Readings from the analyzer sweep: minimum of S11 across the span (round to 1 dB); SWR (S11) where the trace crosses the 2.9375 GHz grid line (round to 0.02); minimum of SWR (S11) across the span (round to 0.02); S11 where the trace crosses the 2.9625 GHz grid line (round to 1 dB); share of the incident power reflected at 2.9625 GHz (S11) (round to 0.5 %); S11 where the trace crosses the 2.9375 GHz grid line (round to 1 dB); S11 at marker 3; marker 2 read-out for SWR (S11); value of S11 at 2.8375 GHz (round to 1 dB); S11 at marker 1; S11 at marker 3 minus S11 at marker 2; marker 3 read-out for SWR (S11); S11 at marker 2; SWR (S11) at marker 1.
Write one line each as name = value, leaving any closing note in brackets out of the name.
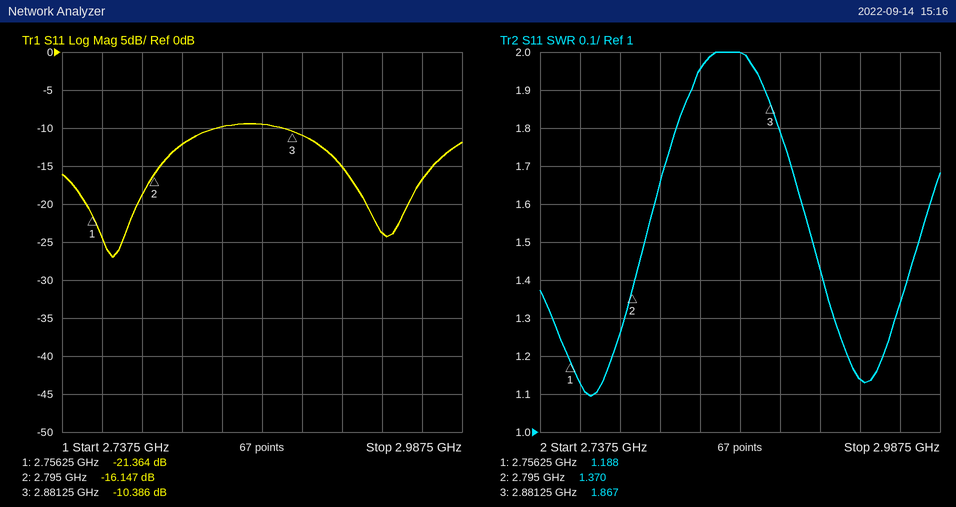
minimum of S11 across the span = -27 dB
SWR (S11) where the trace crosses the 2.9375 GHz grid line = 1.14
minimum of SWR (S11) across the span = 1.10
S11 where the trace crosses the 2.9625 GHz grid line = -17 dB
share of the incident power reflected at 2.9625 GHz (S11) = 2.0 %
S11 where the trace crosses the 2.9375 GHz grid line = -24 dB
S11 at marker 3 = -10.386 dB
marker 2 read-out for SWR = 1.370
value of S11 at 2.8375 GHz = -10 dB
S11 at marker 1 = -21.364 dB
S11 at marker 3 minus S11 at marker 2 = 5.761 dB
marker 3 read-out for SWR = 1.867
S11 at marker 2 = -16.147 dB
SWR (S11) at marker 1 = 1.188
